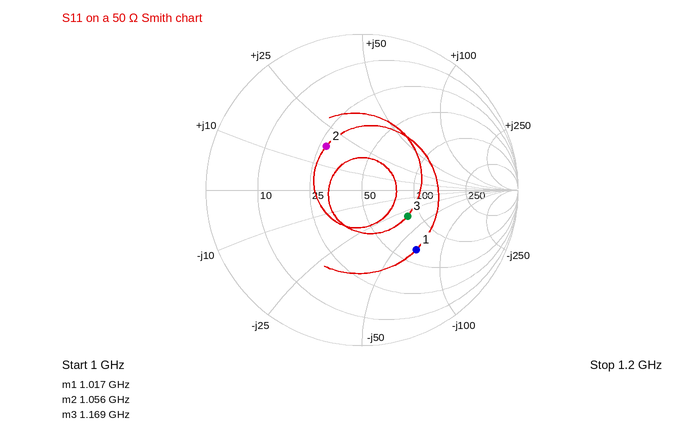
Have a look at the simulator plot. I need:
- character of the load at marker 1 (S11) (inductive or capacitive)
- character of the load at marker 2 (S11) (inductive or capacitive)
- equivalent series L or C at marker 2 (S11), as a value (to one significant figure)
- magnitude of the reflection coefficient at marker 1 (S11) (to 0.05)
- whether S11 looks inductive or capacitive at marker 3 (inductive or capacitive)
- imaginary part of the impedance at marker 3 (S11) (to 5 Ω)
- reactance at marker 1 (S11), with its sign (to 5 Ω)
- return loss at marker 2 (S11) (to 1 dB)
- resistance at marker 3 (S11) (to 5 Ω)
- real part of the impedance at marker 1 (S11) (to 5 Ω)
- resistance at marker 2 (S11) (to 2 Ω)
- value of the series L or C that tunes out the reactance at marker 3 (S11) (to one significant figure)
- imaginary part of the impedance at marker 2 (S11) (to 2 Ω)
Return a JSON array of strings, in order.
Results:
["capacitive", "inductive", "3 nH", "0.50", "capacitive", "-30 Ω", "-65 Ω", "9 dB", "85 Ω", "65 Ω", "28 Ω", "4 nH", "+18 Ω"]
